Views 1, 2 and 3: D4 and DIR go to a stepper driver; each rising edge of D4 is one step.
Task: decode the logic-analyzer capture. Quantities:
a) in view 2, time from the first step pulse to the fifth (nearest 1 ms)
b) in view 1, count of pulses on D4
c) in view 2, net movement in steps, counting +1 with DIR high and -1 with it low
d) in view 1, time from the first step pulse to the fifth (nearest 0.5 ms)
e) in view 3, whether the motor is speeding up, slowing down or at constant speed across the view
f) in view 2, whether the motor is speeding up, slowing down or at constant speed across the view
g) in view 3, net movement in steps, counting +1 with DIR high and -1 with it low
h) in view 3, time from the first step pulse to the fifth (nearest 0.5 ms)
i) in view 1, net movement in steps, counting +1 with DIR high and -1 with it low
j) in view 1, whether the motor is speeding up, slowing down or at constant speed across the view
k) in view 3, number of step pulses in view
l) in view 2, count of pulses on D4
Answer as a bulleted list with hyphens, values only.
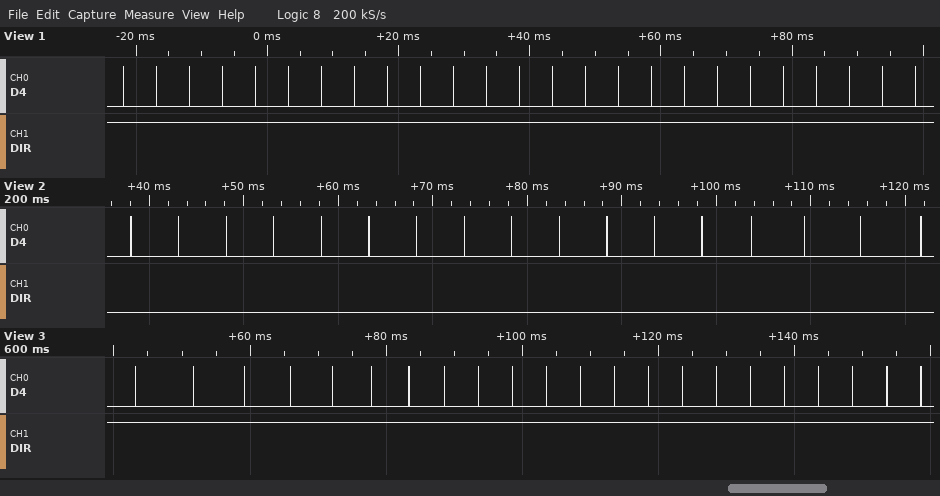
- 20 ms
- 25
- -17
- 20.0 ms
- speeding up
- slowing down
- +22
- 29.0 ms
- +25
- constant speed
- 22
- 17
